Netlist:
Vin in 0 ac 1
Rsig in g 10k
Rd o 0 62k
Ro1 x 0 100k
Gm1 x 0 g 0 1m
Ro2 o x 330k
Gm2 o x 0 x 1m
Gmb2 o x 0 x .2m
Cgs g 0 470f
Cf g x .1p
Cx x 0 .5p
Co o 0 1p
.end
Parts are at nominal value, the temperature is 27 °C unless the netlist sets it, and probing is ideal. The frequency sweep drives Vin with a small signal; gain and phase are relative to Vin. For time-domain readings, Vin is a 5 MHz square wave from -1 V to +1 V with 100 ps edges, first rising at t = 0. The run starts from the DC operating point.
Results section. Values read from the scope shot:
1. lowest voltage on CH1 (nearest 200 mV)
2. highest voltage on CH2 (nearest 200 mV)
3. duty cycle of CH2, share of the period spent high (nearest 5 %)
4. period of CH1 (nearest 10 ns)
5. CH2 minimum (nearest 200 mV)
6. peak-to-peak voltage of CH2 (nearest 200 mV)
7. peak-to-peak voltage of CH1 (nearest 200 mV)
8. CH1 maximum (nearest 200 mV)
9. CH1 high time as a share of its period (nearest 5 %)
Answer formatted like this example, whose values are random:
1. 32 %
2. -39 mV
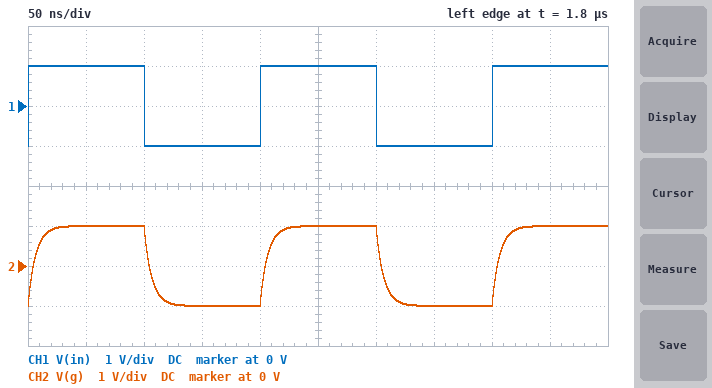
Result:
1. -1.0 V
2. 1.0 V
3. 50 %
4. 200 ns
5. -1.0 V
6. 2.0 V
7. 2.0 V
8. 1.0 V
9. 50 %
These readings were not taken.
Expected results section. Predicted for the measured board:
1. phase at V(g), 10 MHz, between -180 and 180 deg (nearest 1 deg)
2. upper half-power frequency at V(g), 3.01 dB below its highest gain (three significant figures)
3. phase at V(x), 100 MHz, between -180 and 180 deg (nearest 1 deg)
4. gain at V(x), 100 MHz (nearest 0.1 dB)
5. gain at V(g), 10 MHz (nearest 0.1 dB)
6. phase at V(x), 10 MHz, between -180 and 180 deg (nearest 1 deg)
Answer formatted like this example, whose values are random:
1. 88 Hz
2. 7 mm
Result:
1. -22 deg
2. 24.1 MHz
3. 85 deg
4. -14.6 dB
5. -0.7 dB
6. 153 deg
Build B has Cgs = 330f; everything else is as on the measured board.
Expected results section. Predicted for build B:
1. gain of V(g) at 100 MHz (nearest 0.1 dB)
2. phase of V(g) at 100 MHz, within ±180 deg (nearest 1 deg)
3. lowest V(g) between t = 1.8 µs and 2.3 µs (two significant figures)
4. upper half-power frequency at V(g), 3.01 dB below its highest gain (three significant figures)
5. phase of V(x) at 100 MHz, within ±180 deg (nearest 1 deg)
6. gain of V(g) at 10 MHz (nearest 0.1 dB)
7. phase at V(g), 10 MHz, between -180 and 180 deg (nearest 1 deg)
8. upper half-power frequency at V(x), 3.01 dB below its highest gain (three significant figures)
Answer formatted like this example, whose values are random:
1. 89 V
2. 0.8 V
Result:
1. -10.6 dB
2. -70 deg
3. -1.0 V
4. 30.5 MHz
5. 89 deg
6. -0.5 dB
7. -18 deg
8. 19.7 MHz
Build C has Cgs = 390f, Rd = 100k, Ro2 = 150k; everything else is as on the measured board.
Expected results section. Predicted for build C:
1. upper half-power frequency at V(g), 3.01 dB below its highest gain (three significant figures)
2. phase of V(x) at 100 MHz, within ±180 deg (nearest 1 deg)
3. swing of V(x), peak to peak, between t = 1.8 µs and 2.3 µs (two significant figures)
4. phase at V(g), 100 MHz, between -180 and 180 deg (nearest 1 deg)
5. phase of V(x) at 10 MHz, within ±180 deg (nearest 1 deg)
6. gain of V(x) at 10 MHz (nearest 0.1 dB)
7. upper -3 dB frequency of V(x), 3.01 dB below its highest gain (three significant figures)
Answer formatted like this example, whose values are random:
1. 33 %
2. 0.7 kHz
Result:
1. 27.3 MHz
2. 87 deg
3. 2.1 V
4. -72 deg
5. 152 deg
6. -2.1 dB
7. 2.90 MHz
